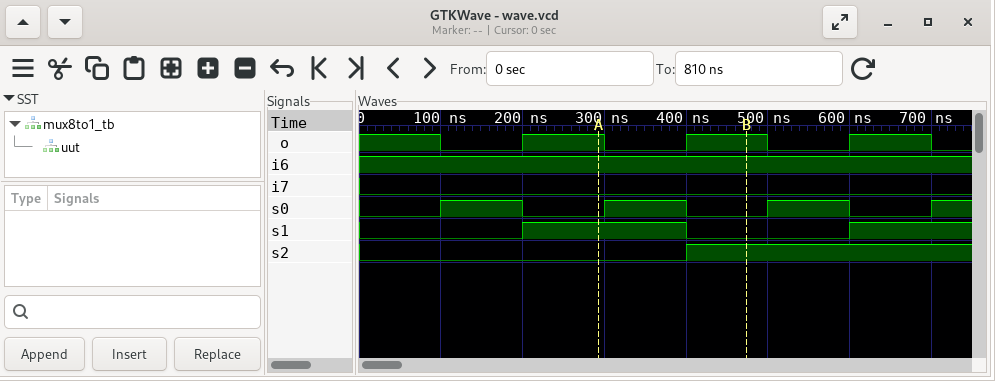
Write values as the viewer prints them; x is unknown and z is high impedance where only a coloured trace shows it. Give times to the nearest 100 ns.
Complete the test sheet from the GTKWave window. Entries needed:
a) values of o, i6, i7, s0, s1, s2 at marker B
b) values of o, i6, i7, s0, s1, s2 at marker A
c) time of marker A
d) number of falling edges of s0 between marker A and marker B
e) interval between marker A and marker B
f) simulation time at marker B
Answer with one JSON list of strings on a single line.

["o=1, i6=1, i7=0, s0=0, s1=0, s2=1", "o=1, i6=1, i7=0, s0=0, s1=1, s2=0", "300 ns", "1", "200 ns", "500 ns"]
